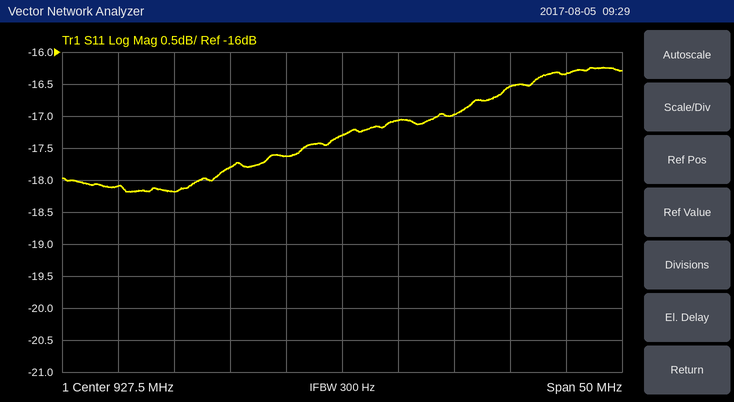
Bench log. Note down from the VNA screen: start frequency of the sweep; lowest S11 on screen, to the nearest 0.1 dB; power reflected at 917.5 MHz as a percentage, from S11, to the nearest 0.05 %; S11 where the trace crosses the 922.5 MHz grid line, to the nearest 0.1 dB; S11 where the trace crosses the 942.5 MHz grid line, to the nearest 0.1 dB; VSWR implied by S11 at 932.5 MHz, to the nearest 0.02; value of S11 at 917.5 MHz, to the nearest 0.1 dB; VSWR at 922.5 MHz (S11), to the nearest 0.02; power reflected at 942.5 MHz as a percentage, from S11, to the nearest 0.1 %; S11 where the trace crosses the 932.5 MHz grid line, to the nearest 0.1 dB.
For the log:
902.5 MHz
-18.2 dB
1.65 %
-17.6 dB
-16.5 dB
1.32
-17.8 dB
1.30
2.2 %
-17.1 dB
